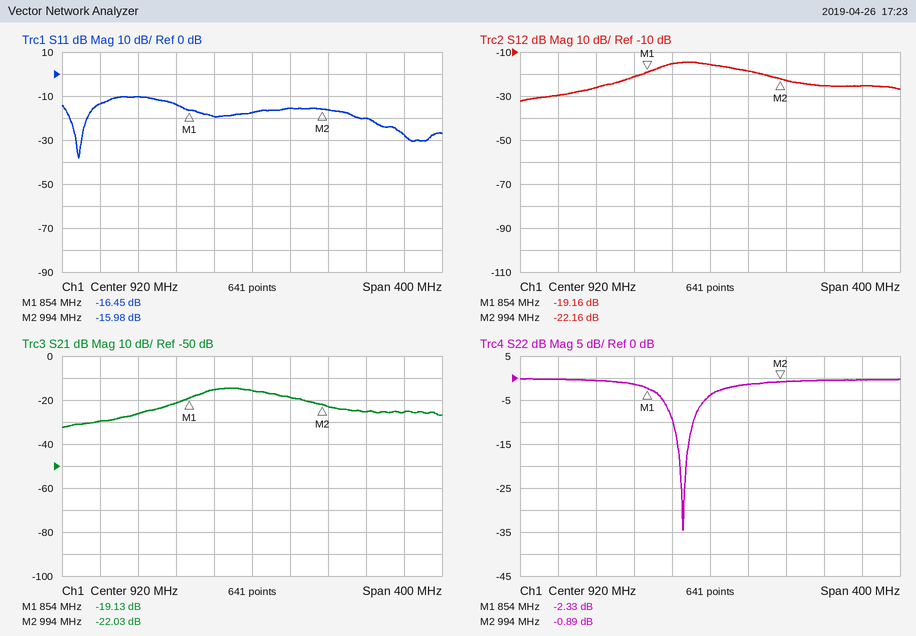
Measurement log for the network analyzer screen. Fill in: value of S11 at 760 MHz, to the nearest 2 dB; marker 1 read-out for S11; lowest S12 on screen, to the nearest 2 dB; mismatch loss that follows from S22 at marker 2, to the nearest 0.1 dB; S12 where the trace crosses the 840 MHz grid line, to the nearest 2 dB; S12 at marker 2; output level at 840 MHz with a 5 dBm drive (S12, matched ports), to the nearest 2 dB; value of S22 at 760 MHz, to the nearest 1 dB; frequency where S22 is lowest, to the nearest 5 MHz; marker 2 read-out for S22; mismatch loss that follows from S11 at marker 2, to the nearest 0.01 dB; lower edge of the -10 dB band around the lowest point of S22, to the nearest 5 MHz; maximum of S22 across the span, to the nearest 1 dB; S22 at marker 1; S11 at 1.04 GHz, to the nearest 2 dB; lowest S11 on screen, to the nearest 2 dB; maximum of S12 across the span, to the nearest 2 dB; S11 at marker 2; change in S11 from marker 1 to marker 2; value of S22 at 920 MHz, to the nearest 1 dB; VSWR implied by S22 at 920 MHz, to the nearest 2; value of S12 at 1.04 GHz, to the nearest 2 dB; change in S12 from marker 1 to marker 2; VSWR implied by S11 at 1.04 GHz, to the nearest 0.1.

-14 dB
-16.45 dB
-32 dB
7.3 dB
-22 dB
-22.16 dB
-16 dBm
0 dB
890 MHz
-0.89 dB
0.11 dB
880 MHz
0 dB
-2.33 dB
-20 dB
-38 dB
-14 dB
-15.98 dB
0.47 dB
-4 dB
4
-26 dB
-3.00 dB
1.2
